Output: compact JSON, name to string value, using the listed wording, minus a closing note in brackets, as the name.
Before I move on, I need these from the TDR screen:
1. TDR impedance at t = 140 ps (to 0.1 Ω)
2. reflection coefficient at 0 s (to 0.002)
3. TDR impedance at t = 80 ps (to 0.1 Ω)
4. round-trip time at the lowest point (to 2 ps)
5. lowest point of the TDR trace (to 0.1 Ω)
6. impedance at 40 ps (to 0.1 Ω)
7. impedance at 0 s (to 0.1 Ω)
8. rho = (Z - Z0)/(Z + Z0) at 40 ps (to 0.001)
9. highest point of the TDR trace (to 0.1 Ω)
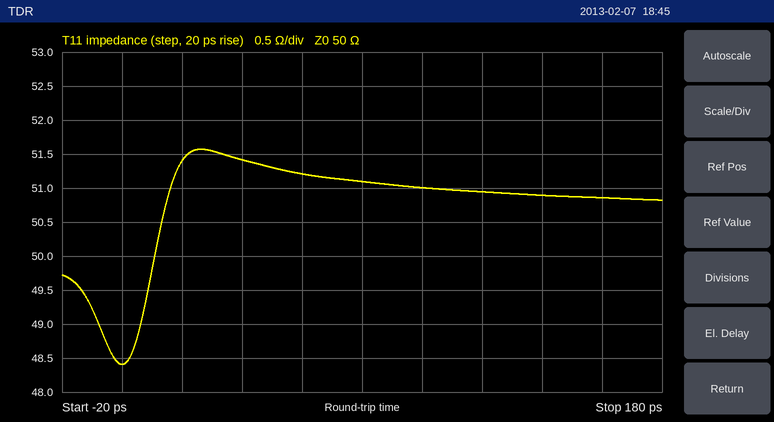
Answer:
{"TDR impedance at t = 140 ps": "50.9 Ω", "reflection coefficient at 0 s": "-0.016", "TDR impedance at t = 80 ps": "51.1 Ω", "round-trip time at the lowest point": "0 ps", "lowest point of the TDR trace": "48.4 Ω", "impedance at 40 ps": "51.4 Ω", "impedance at 0 s": "48.4 Ω", "rho = (Z - Z0)/(Z + Z0) at 40 ps": "+0.014", "highest point of the TDR trace": "51.6 Ω"}
